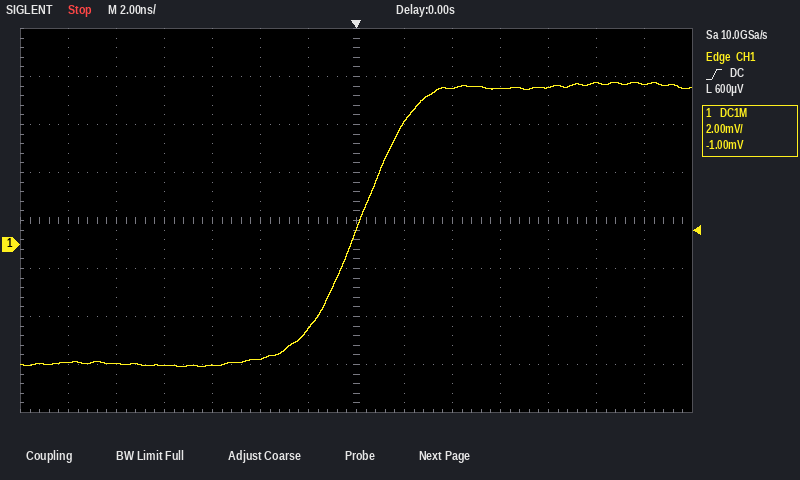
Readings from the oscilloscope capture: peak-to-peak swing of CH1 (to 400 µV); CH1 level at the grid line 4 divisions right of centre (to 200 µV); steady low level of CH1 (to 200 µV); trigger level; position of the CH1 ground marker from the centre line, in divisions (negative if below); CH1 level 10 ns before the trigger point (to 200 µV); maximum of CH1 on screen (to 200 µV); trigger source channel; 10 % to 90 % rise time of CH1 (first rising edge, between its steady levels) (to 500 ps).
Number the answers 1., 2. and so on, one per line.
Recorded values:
1. 12.0 mV
2. 6.6 mV
3. -5.0 mV
4. 600 µV
5. -0.5 div
6. -5.0 mV
7. 6.8 mV
8. CH1
9. 4.5 ns
